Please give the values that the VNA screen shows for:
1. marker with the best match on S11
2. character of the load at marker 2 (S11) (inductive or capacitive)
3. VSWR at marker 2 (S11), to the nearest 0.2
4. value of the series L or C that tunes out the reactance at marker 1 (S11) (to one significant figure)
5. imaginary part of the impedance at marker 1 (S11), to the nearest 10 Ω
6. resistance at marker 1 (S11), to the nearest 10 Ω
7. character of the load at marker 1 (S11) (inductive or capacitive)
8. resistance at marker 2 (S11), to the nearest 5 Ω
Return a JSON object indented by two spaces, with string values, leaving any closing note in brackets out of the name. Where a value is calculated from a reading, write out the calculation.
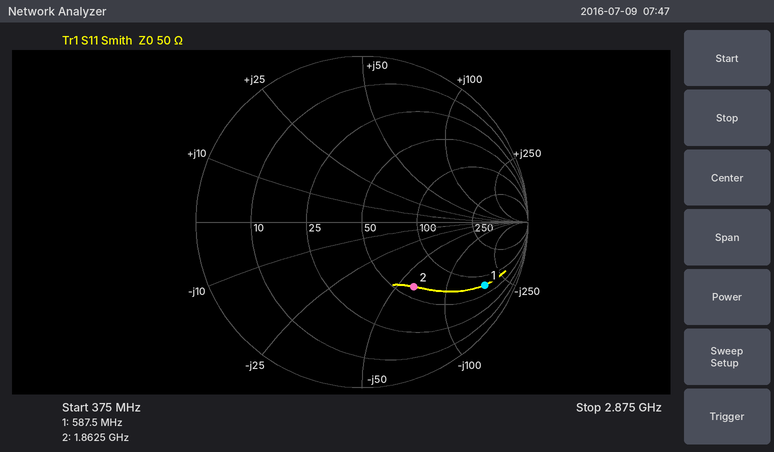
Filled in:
{
  "marker with the best match on S11": "marker 2",
  "character of the load at marker 2 (S11)": "capacitive",
  "VSWR at marker 2 (S11), to the nearest 0.2": "3.0",
  "value of the series L or C that tunes out the reactance at marker 1 (S11)": "L = 180 Ω/(2π × 587.5 MHz) ≈ 48.8 nH, so 50 nH to one significant figure",
  "imaginary part of the impedance at marker 1 (S11), to the nearest 10 Ω": "-180 Ω",
  "resistance at marker 1 (S11), to the nearest 10 Ω": "70 Ω",
  "character of the load at marker 1 (S11)": "capacitive",
  "resistance at marker 2 (S11), to the nearest 5 Ω": "60 Ω"
}
